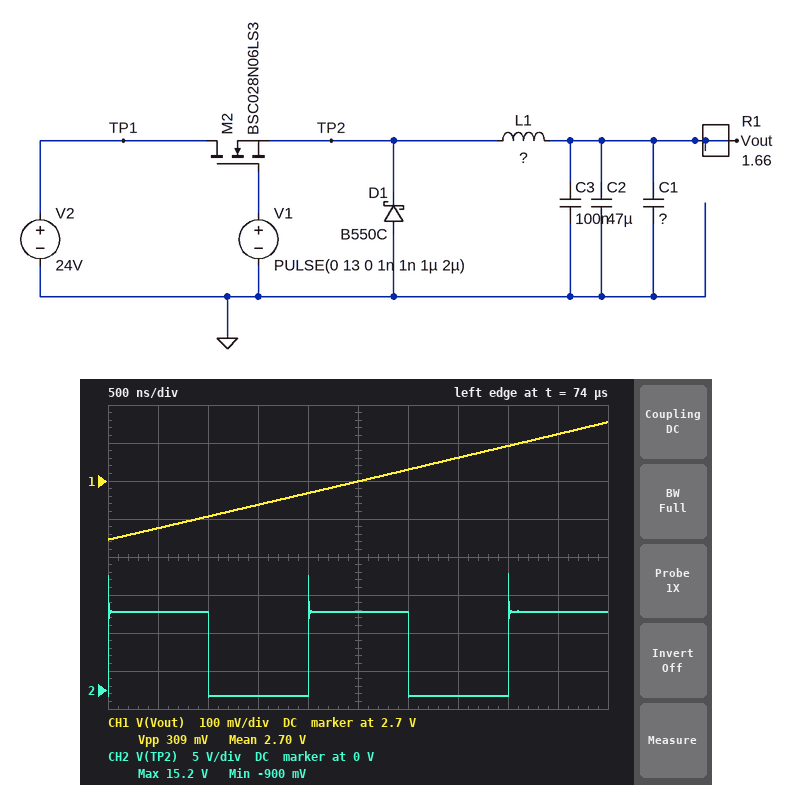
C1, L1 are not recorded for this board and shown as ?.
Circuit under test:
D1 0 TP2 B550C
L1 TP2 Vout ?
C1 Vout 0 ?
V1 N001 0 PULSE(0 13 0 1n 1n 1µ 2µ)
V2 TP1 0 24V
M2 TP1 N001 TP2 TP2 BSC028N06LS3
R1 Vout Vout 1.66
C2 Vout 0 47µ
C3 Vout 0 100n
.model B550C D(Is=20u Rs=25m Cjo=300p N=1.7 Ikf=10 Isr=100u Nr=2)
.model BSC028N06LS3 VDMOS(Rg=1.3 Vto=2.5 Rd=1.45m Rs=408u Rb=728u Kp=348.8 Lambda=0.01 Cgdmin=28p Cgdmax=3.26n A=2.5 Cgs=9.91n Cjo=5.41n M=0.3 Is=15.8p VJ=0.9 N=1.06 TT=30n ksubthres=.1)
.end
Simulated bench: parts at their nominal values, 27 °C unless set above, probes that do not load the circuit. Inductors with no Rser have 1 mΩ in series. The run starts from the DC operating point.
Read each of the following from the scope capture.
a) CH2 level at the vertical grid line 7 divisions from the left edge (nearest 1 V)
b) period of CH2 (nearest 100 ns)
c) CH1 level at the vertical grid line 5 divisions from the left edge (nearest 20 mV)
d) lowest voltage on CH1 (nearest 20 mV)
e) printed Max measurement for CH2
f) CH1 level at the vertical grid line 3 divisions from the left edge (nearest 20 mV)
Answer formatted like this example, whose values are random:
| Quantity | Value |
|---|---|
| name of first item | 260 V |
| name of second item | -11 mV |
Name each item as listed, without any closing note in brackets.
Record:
| Quantity | Value |
|---|---|
| CH2 level at the vertical grid line 7 divisions from the left edge | -1 V |
| period of CH2 | 2.0 µs |
| CH1 level at the vertical grid line 5 divisions from the left edge | 2.70 V |
| lowest voltage on CH1 | 2.54 V |
| printed Max measurement for CH2 | 15.2 V |
| CH1 level at the vertical grid line 3 divisions from the left edge | 2.64 V |
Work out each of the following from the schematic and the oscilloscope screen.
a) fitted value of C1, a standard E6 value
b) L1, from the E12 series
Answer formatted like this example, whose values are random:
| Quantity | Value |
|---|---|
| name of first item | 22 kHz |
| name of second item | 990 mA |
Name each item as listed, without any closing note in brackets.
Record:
| Quantity | Value |
|---|---|
| fitted value of C1, a standard E6 value | 100 µF |
| L1, from the E12 series | 33 µH |
